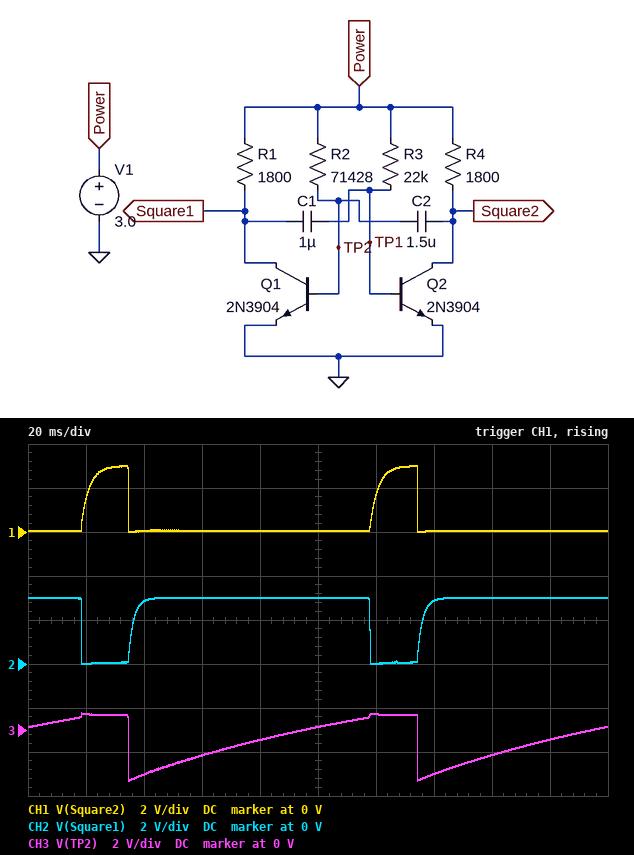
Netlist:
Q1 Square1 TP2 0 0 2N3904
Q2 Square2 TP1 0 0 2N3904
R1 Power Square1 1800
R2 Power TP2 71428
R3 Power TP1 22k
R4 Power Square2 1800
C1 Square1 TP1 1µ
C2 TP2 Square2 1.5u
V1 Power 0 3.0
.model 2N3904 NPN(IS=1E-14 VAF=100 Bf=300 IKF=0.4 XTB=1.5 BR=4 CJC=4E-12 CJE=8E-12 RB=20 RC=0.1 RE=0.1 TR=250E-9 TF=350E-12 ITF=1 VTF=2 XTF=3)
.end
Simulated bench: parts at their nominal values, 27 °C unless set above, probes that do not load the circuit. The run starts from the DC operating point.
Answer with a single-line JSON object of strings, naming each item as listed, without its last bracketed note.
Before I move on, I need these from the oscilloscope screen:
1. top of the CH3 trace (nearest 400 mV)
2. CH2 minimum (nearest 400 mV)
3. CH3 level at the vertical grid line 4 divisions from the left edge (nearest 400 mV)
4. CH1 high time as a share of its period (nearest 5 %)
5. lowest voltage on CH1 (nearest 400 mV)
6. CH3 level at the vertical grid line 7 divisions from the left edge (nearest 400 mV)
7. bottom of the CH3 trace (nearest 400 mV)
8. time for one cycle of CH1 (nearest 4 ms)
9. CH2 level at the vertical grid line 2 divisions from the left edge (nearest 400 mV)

{"top of the CH3 trace": "800 mV", "CH2 minimum": "0 V", "CH3 level at the vertical grid line 4 divisions from the left edge": "-400 mV", "CH1 high time as a share of its period": "15 %", "lowest voltage on CH1": "0 V", "CH3 level at the vertical grid line 7 divisions from the left edge": "-2.0 V", "bottom of the CH3 trace": "-2.4 V", "time for one cycle of CH1": "100 ms", "CH2 level at the vertical grid line 2 divisions from the left edge": "2.8 V"}
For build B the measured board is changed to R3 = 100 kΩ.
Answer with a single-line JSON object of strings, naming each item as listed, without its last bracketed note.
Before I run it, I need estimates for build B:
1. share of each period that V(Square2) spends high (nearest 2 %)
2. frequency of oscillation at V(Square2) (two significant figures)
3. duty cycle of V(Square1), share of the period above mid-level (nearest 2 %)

{"share of each period that V(Square2) spends high": "48 %", "frequency of oscillation at V(Square2)": "6.4 Hz", "duty cycle of V(Square1), share of the period above mid-level": "50 %"}
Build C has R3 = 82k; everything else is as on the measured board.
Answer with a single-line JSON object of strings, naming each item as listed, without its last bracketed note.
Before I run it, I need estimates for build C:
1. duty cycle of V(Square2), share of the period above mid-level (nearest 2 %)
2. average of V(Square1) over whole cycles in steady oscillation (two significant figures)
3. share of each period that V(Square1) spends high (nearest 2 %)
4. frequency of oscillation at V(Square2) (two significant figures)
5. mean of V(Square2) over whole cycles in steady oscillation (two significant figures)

{"duty cycle of V(Square2), share of the period above mid-level": "42 %", "average of V(Square1) over whole cycles in steady oscillation": "1.7 V", "share of each period that V(Square1) spends high": "56 %", "frequency of oscillation at V(Square2)": "7.0 Hz", "mean of V(Square2) over whole cycles in steady oscillation": "1.3 V"}
